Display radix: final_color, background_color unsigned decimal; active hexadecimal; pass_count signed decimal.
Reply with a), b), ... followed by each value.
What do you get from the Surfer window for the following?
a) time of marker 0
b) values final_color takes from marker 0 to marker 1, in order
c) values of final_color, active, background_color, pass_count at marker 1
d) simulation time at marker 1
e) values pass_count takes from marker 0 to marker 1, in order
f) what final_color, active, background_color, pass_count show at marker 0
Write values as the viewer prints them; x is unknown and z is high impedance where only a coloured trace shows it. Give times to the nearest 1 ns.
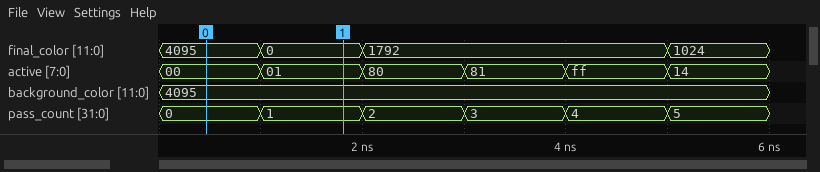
a) 0 ns
b) 4095, 0
c) final_color=0, active=01, background_color=4095, pass_count=1
d) 2 ns
e) 0, 1
f) final_color=4095, active=00, background_color=4095, pass_count=0
